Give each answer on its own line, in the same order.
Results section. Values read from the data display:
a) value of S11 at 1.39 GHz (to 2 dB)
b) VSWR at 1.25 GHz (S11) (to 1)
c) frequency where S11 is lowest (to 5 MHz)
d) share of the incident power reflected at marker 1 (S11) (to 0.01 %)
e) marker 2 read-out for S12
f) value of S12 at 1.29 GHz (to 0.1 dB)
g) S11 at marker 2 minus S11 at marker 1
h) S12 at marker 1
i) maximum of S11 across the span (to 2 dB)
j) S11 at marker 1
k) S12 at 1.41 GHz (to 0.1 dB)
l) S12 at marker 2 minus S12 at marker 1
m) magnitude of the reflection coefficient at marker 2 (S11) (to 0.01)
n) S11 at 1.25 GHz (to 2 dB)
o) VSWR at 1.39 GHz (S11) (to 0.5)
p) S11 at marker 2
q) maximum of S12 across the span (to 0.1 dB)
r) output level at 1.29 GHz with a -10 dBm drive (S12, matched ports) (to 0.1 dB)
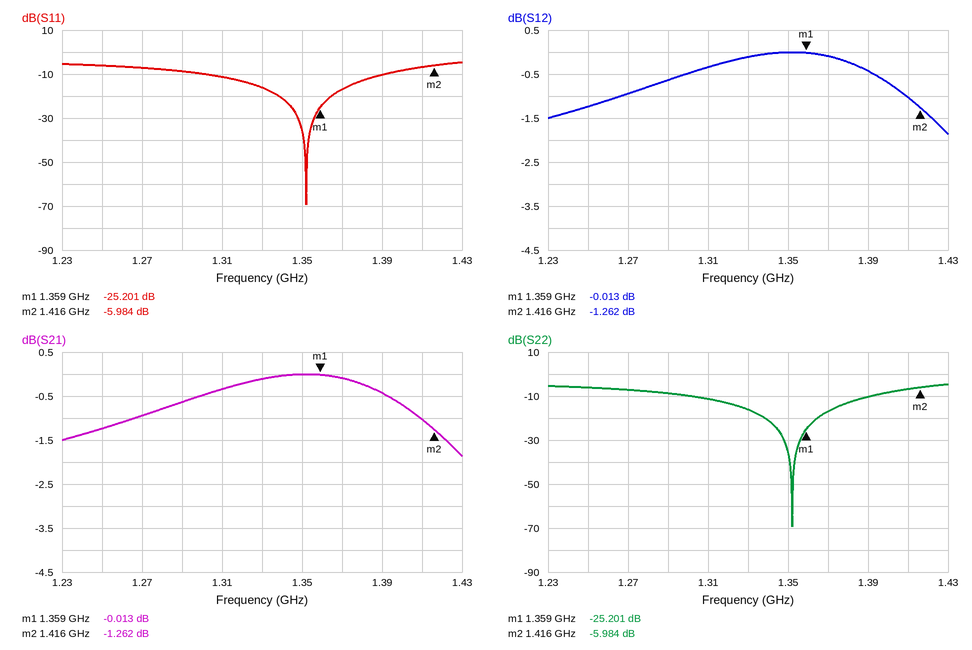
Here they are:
-10 dB
3
1.350 GHz
0.30 %
-1.262 dB
-0.6 dB
19.217 dB
-0.013 dB
-4 dB
-25.201 dB
-1.0 dB
-1.249 dB
0.50
-6 dB
2.0
-5.984 dB
0.0 dB
-10.6 dBm
